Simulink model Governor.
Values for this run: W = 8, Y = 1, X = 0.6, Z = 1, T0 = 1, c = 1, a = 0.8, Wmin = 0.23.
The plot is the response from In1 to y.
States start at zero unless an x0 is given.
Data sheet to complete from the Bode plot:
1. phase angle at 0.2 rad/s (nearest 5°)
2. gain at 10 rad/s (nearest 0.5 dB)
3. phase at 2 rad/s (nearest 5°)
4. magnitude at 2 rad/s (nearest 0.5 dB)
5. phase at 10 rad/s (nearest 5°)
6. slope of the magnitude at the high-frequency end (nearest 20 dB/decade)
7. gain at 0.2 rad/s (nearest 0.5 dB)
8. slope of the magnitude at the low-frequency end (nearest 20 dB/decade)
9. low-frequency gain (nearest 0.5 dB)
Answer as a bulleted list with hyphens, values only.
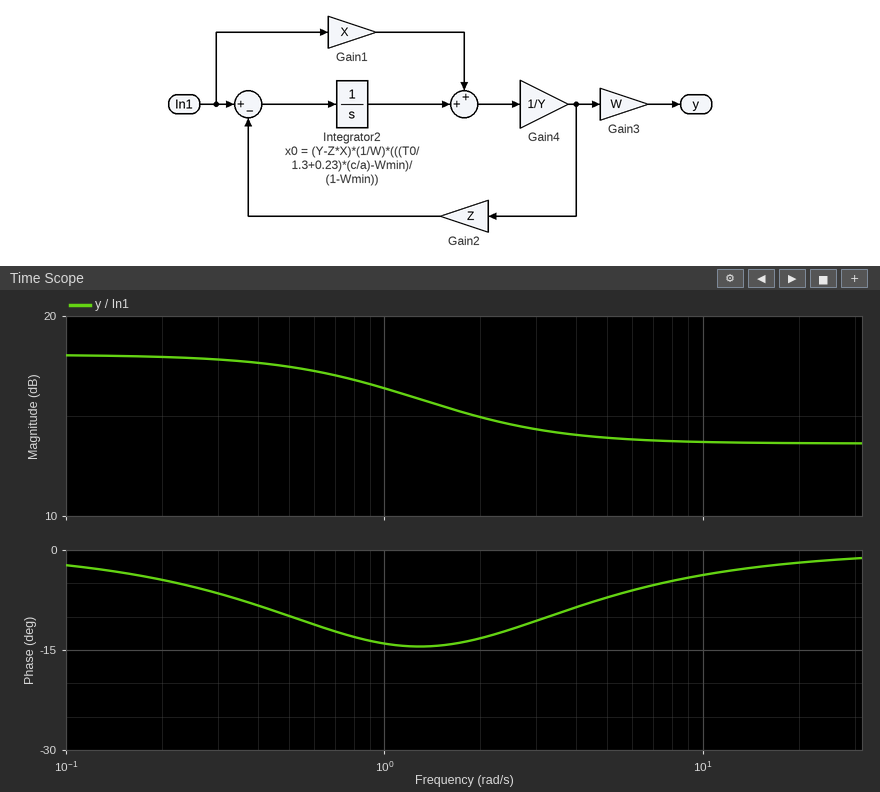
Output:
- -5°
- 13.5 dB
- -15°
- 15.0 dB
- -5°
- 0 dB/decade
- 18.0 dB
- 0 dB/decade
- 18.0 dB
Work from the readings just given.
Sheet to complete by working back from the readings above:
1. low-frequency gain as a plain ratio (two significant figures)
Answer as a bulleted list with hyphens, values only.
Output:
- 7.9
